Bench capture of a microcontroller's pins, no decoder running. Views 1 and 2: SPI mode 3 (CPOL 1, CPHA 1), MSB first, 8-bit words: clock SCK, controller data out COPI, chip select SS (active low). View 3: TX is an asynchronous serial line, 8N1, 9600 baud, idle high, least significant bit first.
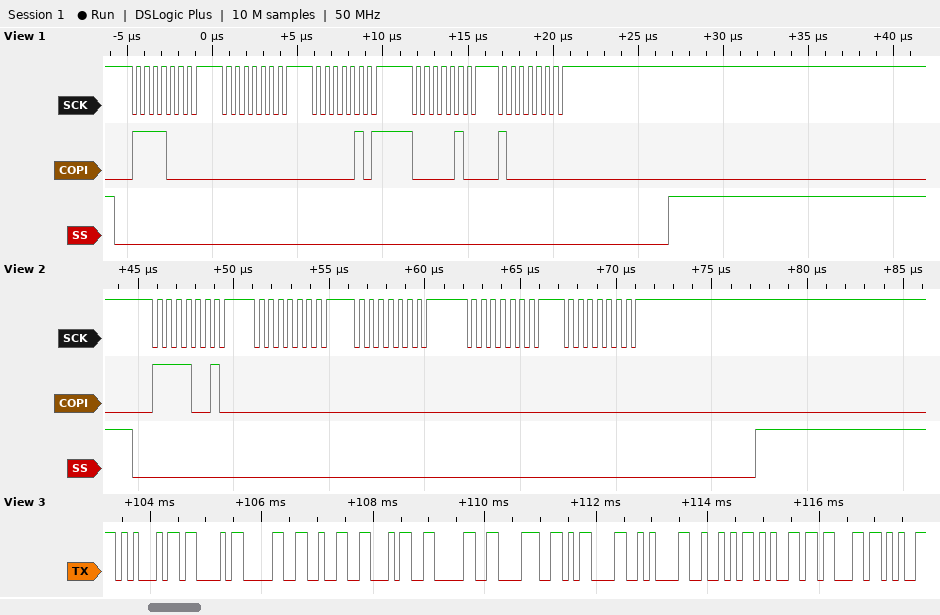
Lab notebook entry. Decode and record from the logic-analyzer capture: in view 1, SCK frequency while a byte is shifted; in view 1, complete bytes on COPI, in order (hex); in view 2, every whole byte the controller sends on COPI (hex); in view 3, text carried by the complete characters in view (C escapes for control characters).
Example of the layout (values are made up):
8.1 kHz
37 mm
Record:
2 MHz
F0 00 05 04 80
F2 00 00 00 00
"EC02408\r\nRec"
